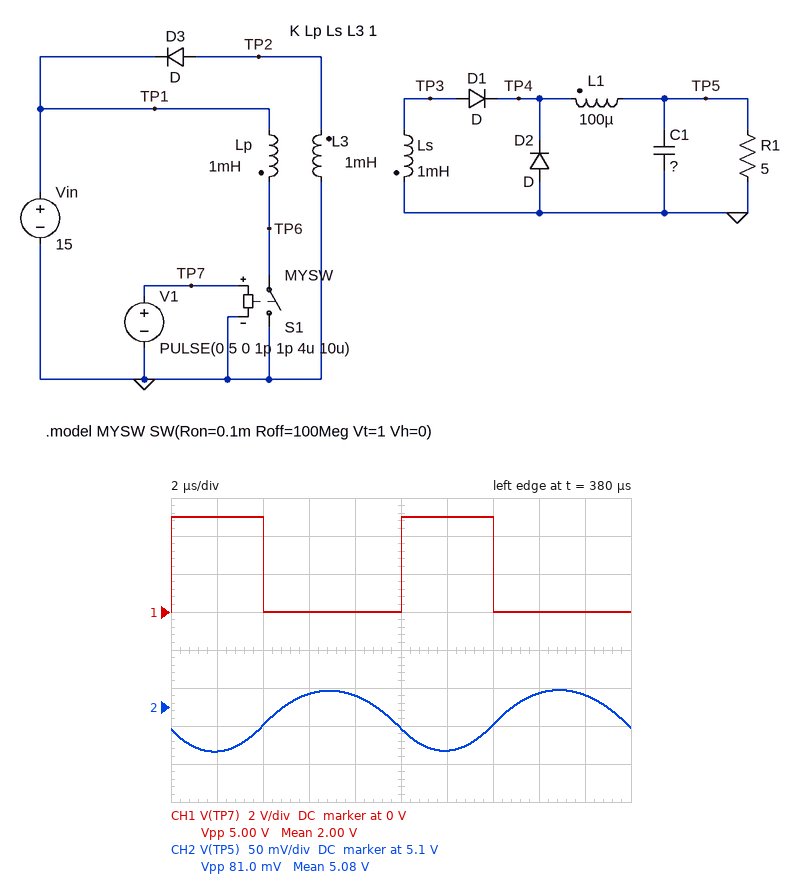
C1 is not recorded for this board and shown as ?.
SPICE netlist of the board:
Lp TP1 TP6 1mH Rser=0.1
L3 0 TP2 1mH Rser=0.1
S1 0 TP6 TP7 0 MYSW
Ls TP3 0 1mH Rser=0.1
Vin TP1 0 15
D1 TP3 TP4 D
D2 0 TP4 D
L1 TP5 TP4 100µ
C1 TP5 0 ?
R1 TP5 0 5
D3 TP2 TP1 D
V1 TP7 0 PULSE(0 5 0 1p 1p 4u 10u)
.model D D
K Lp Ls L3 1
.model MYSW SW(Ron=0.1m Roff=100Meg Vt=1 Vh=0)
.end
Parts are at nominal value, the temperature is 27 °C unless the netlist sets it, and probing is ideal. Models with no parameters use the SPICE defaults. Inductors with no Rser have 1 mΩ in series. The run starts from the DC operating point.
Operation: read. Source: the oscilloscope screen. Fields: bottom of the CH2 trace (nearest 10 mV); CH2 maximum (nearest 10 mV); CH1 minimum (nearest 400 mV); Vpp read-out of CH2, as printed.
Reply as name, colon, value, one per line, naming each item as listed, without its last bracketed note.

bottom of the CH2 trace: 5.04 V
CH2 maximum: 5.12 V
CH1 minimum: 0 V
Vpp read-out of CH2, as printed: 81.0 mV
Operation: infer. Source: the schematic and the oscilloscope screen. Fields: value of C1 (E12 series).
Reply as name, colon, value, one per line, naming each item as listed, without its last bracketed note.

value of C1: 5.6 µF
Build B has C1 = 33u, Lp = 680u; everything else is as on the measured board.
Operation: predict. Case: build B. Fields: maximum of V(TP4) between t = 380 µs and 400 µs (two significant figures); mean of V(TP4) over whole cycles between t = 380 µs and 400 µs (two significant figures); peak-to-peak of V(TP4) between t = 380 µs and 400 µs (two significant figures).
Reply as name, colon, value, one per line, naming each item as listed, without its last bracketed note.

maximum of V(TP4) between t = 380 µs and 400 µs: 17 V
mean of V(TP4) over whole cycles between t = 380 µs and 400 µs: 6.3 V
peak-to-peak of V(TP4) between t = 380 µs and 400 µs: 18 V
